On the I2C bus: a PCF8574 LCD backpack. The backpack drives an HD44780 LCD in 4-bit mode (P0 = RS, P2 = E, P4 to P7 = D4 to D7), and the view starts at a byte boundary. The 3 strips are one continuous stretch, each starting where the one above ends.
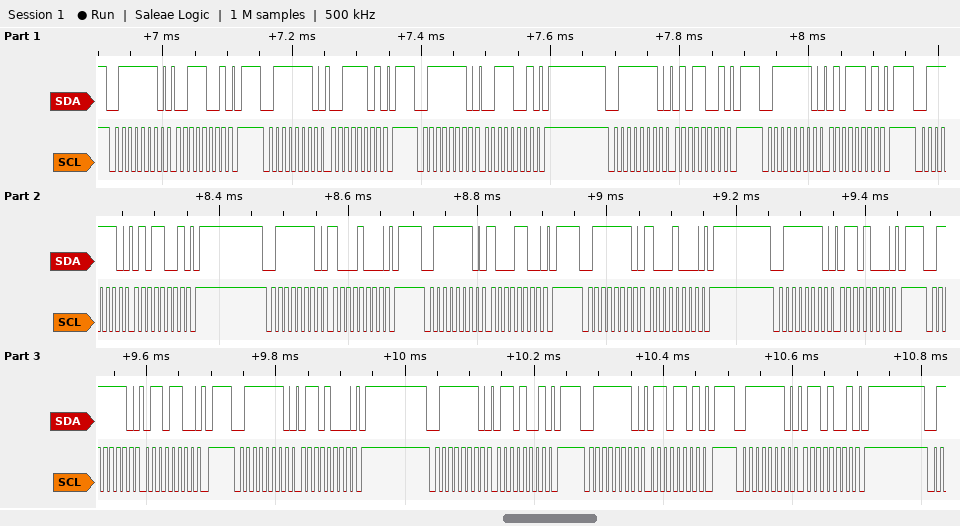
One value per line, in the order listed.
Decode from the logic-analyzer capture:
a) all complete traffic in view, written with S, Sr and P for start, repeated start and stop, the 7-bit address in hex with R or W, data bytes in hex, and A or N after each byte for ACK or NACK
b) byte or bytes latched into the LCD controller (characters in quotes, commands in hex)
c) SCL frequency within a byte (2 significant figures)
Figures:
S 3FW A 39 A P S 3FW A 3D A P S 3FW A 39 A P S 3FW A 59 A P S 3FW A 5D A P S 3FW A 59 A P S 3FW A 88 A P S 3FW A 8C A P S 3FW A 88 A P S 3FW A 68 A P S 3FW A 6C A P S 3FW A 68 A P S 3FW A 69 A P S 3FW A 6D A P S 3FW A 69 A P
'5' 0x86
100 kHz
